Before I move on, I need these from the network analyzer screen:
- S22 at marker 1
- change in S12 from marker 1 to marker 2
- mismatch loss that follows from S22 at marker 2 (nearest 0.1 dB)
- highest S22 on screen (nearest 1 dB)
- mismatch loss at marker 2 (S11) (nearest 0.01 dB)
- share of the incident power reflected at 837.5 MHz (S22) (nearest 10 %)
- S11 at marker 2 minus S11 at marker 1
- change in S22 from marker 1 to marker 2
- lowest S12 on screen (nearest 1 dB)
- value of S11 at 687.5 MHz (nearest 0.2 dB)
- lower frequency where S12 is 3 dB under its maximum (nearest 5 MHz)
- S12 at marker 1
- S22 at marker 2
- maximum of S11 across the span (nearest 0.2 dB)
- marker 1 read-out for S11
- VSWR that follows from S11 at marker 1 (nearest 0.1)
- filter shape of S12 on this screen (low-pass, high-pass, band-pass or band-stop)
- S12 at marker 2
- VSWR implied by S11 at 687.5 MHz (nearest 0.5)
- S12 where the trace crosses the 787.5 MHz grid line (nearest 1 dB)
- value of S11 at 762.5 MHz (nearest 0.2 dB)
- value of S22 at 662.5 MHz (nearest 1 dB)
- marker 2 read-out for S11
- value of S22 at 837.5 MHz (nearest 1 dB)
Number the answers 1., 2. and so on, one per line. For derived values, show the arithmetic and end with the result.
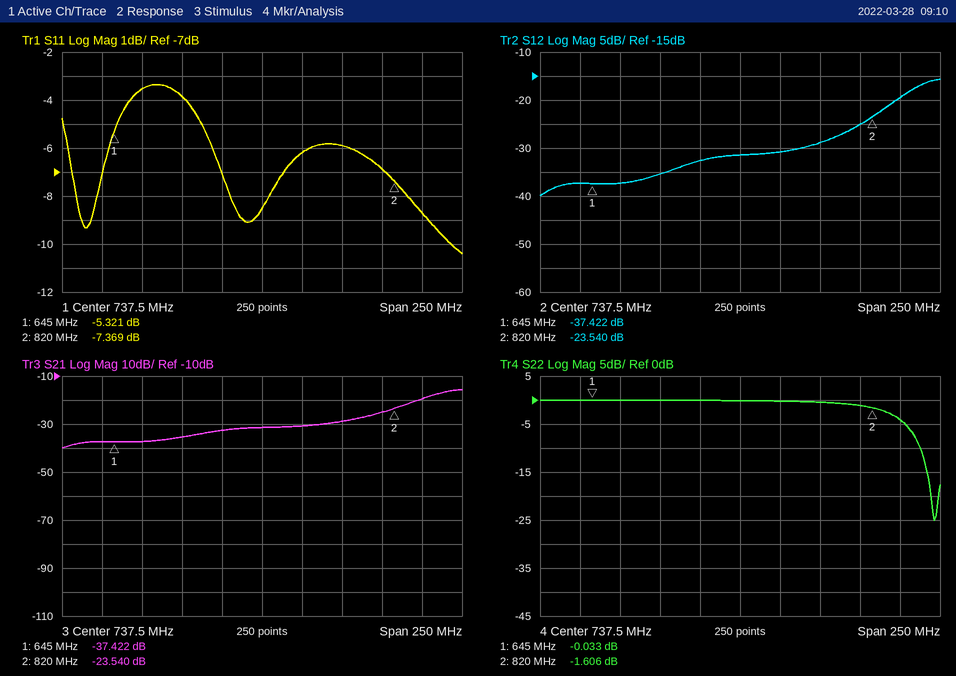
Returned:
1. -0.033 dB
2. -23.54 − (-37.422) = 13.882 dB
3. −10 log10(1 − 10^(-1.606/10)) ≈ 5.1 dB
4. 0 dB
5. −10 log10(1 − 10^(-7.369/10)) ≈ 0.88 dB
6. 10^(-4/10) ≈ 40 %
7. -7.369 − (-5.321) = -2.048 dB
8. -1.606 − (-0.033) = -1.573 dB
9. -40 dB
10. -3.8 dB
11. 840 MHz
12. -37.422 dB
13. -1.606 dB
14. -3.4 dB
15. -5.321 dB
16. (1 + 0.5419)/(1 − 0.5419) ≈ 3.4
17. high-pass
18. -23.540 dB
19. |Γ| = 10^(-3.8/20) = 0.6457; VSWR = (1 + 0.6457)/(1 − 0.6457) ≈ 4.64, so 4.5 to the nearest 0.5
20. -29 dB
21. -6.2 dB
22. 0 dB
23. -7.369 dB
24. -4 dB
